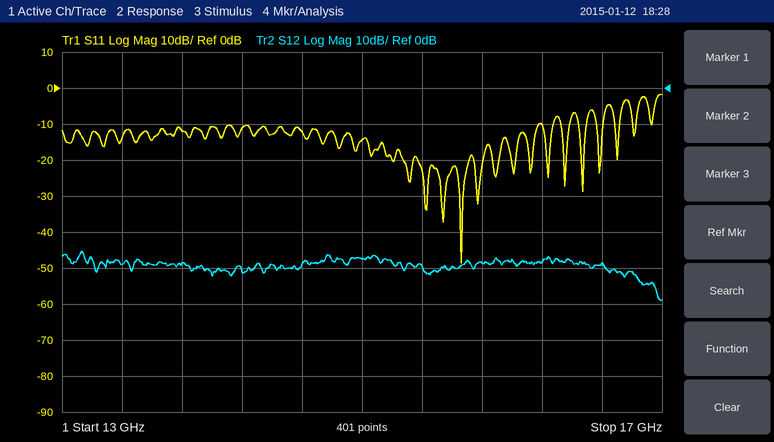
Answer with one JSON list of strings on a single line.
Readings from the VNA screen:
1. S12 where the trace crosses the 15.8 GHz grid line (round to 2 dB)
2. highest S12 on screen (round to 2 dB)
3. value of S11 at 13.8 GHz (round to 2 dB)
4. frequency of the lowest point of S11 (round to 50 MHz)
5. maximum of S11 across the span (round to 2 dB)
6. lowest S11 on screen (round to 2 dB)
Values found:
["-48 dB", "-46 dB", "-12 dB", "15.65 GHz", "-2 dB", "-48 dB"]
